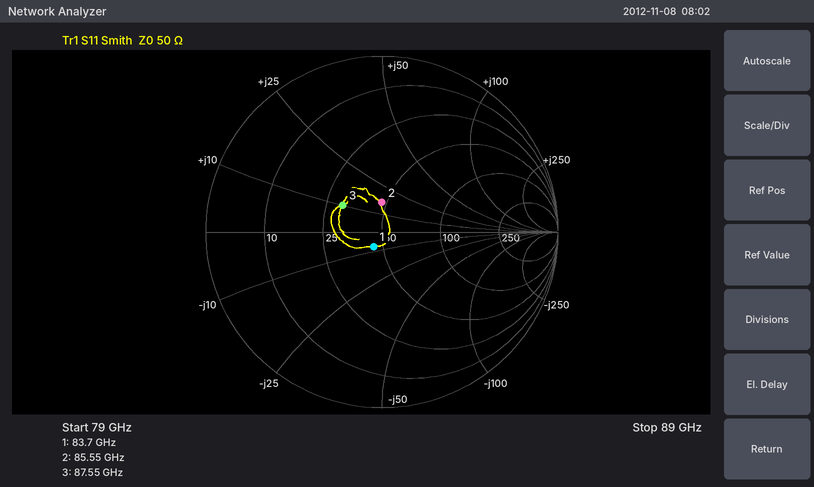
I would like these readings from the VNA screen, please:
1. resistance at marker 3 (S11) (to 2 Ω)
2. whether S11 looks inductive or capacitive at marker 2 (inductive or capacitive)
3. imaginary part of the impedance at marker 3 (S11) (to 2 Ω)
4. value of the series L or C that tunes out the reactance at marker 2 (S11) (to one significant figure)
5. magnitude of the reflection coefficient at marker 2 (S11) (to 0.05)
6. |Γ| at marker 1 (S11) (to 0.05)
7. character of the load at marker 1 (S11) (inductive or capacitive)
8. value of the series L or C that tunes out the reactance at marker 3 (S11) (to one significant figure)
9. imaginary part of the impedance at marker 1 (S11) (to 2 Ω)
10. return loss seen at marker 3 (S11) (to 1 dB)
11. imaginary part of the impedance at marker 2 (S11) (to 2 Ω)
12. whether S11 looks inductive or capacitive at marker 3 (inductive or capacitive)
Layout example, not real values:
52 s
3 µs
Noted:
30 Ω
inductive
+10 Ω
100 fF
0.15
0.10
capacitive
200 fF
-8 Ω
11 dB
+16 Ω
inductive
